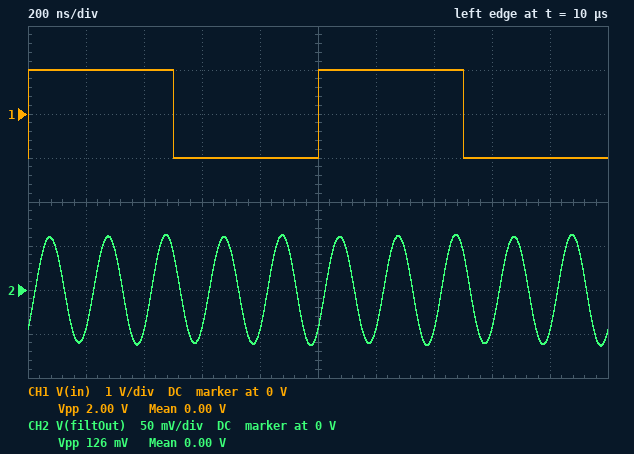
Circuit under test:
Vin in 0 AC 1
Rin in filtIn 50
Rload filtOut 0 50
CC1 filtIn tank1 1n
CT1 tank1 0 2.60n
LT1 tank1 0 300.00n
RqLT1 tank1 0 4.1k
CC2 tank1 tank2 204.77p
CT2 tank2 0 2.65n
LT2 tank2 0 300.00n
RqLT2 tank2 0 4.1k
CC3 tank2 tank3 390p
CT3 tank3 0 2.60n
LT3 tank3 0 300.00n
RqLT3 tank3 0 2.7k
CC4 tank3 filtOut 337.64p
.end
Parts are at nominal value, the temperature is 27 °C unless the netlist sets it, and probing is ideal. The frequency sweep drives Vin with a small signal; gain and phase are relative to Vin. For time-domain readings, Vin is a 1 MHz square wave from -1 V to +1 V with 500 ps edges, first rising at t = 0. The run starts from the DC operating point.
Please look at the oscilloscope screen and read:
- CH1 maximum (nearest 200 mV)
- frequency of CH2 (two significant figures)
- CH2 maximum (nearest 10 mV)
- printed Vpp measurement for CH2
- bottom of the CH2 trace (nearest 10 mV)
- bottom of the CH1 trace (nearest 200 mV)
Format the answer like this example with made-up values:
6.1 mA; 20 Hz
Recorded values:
1.0 V; 5.0 MHz; 60 mV; 126 mV; -60 mV; -1.0 V
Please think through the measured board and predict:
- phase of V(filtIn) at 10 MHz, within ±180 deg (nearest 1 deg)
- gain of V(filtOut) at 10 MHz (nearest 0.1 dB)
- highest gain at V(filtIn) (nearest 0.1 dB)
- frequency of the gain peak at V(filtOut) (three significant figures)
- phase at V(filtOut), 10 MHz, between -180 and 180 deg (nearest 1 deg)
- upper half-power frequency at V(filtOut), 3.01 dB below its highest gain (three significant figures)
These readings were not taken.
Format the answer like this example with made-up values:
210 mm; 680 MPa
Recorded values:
-64 deg; -56.0 dB; 0 dB; 5.43 MHz; -16 deg; 5.54 MHz
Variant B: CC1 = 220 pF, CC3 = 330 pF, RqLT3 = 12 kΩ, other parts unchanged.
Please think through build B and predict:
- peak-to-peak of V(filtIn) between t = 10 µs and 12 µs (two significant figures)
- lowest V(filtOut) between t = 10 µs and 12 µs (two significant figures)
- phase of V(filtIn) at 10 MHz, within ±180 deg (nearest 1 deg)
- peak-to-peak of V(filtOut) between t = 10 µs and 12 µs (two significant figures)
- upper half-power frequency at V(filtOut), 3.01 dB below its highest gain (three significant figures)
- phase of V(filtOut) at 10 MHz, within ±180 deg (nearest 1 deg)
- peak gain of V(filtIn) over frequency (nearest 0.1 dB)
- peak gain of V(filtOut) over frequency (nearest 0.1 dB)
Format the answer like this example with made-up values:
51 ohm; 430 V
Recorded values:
2.1 V; -46 mV; -32 deg; 91 mV; 5.57 MHz; 16 deg; 0 dB; -6.6 dB
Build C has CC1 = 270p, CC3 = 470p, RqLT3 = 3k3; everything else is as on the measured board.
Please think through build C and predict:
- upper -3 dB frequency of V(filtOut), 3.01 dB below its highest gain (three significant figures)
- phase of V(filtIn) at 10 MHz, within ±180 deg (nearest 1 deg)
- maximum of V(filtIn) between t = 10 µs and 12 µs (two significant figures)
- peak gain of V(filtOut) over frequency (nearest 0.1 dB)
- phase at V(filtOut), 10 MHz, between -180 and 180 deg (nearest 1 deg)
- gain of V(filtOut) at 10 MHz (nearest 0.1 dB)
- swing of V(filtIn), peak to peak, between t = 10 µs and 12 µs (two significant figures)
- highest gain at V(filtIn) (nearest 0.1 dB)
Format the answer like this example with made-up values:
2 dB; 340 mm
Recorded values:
5.57 MHz; -37 deg; 1.1 V; -7.1 dB; 11 deg; -58.4 dB; 2.2 V; 0 dB
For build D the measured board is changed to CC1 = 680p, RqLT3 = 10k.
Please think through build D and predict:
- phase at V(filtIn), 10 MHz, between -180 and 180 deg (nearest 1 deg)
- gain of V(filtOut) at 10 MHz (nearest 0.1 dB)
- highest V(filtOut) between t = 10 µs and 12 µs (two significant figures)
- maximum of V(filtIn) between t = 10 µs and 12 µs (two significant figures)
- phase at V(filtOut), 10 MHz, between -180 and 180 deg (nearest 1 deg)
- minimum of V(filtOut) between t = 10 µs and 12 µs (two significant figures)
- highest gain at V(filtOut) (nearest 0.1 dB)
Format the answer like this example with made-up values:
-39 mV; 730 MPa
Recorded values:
-58 deg; -56.5 dB; 67 mV; 1.2 V; -10 deg; -67 mV; -6.7 dB
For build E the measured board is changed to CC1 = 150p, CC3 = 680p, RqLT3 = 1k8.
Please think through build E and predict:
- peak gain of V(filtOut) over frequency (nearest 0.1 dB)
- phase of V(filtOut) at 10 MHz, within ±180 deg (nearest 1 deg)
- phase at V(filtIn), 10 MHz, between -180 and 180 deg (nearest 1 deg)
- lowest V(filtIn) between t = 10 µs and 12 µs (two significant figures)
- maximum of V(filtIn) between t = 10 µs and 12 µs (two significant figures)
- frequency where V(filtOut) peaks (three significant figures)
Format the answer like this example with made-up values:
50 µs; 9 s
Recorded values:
-7.6 dB; 24 deg; -24 deg; -1.0 V; 1.0 V; 5.28 MHz
